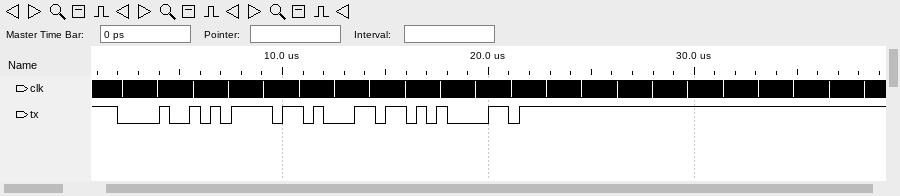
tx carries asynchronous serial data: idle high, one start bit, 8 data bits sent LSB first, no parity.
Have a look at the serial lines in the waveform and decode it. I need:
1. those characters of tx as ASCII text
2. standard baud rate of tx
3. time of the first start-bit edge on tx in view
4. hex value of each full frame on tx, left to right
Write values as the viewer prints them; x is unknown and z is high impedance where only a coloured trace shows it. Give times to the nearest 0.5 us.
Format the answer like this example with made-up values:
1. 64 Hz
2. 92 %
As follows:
1. "Hola"
2. 2000000 baud
3. 2 us
4. 48, 6F, 6C, 61
